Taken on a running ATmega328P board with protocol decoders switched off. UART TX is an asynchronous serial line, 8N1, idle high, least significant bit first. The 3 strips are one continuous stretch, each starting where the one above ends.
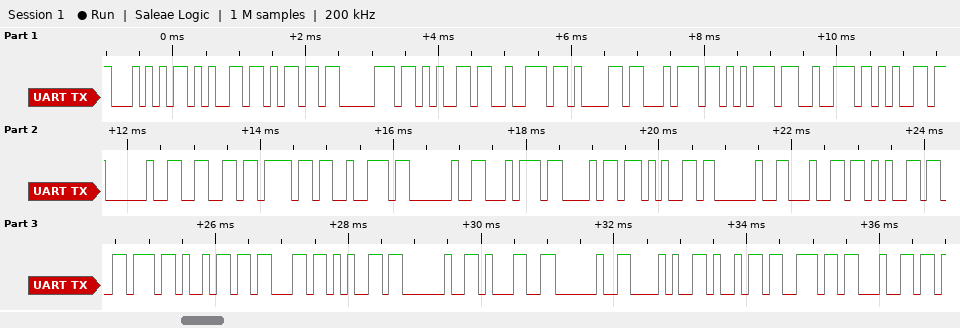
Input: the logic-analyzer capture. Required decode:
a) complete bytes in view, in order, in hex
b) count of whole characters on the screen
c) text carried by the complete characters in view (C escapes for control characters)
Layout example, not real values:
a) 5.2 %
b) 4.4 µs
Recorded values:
a) 54 65 6D 70 65 72 61 74 75 72 65 20 66 6F 72 20 74 68 65 20 64 65 76 69 63 65 20 31 20 28 69 6E 64
b) 33
c) "Temperature for the device 1 (ind"
